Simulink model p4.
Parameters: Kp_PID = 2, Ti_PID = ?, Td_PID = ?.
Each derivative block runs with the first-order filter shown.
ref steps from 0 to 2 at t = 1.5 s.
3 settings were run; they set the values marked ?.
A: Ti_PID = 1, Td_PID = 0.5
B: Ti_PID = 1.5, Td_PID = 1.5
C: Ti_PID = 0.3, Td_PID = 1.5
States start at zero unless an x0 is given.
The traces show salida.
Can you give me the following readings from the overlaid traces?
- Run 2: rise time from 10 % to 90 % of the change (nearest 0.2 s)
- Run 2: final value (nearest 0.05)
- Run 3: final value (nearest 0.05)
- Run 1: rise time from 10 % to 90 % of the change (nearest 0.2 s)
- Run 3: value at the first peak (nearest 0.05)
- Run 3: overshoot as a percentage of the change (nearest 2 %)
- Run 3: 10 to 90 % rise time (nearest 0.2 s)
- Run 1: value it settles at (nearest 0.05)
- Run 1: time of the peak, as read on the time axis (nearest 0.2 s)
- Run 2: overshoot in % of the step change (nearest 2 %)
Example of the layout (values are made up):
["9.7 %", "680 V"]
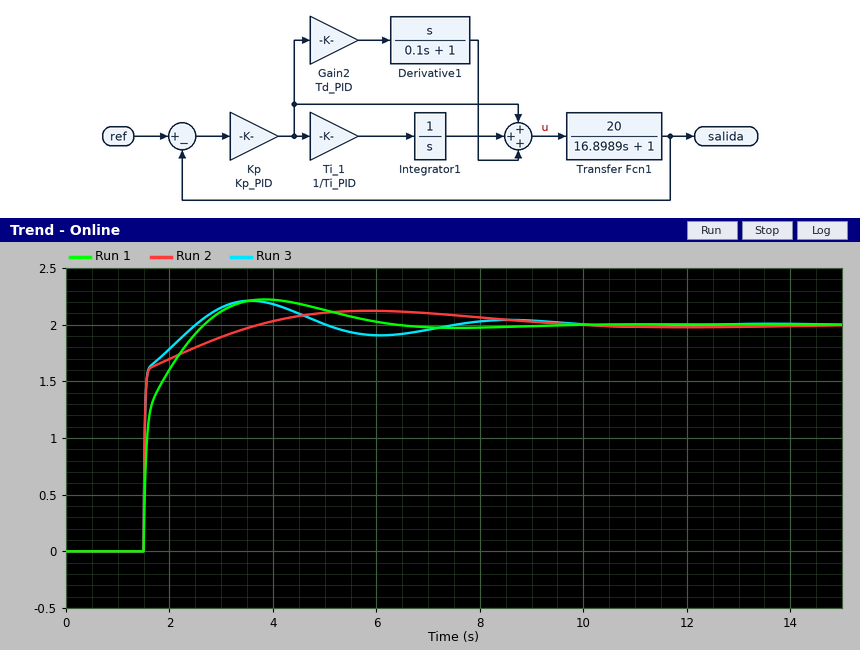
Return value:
["1.0 s", "2.00", "2.00", "0.8 s", "2.20", "10 %", "0.6 s", "2.00", "3.8 s", "6 %"]
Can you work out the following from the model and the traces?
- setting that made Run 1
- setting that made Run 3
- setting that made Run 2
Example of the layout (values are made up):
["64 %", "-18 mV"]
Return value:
["A", "C", "B"]
